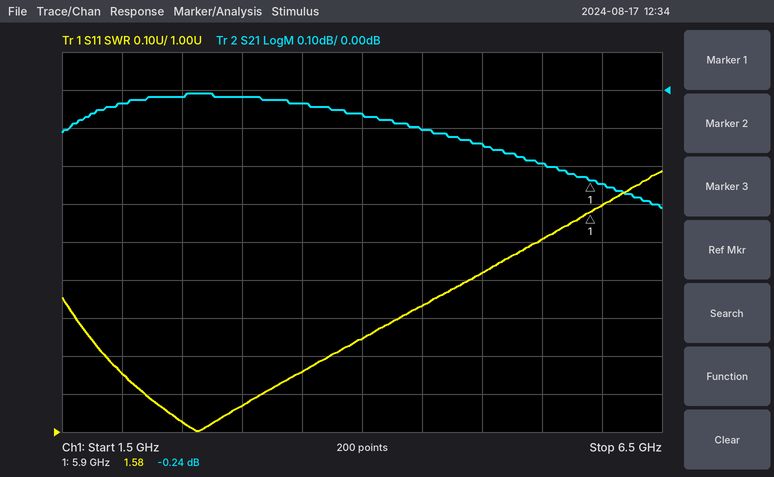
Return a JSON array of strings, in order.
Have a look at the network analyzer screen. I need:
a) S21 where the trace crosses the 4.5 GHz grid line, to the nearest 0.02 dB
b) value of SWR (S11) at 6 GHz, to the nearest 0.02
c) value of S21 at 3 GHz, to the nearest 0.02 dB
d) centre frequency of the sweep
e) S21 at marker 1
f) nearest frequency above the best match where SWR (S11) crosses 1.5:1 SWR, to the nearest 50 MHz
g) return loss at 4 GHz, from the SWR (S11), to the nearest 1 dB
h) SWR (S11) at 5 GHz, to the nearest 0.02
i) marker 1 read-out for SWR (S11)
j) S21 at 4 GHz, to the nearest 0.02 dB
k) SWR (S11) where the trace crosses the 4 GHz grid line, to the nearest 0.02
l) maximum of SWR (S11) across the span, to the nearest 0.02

["-0.10 dB", "1.60", "-0.02 dB", "4 GHz", "-0.24 dB", "5.45 GHz", "19 dB", "1.42", "1.58", "-0.06 dB", "1.24", "1.68"]
